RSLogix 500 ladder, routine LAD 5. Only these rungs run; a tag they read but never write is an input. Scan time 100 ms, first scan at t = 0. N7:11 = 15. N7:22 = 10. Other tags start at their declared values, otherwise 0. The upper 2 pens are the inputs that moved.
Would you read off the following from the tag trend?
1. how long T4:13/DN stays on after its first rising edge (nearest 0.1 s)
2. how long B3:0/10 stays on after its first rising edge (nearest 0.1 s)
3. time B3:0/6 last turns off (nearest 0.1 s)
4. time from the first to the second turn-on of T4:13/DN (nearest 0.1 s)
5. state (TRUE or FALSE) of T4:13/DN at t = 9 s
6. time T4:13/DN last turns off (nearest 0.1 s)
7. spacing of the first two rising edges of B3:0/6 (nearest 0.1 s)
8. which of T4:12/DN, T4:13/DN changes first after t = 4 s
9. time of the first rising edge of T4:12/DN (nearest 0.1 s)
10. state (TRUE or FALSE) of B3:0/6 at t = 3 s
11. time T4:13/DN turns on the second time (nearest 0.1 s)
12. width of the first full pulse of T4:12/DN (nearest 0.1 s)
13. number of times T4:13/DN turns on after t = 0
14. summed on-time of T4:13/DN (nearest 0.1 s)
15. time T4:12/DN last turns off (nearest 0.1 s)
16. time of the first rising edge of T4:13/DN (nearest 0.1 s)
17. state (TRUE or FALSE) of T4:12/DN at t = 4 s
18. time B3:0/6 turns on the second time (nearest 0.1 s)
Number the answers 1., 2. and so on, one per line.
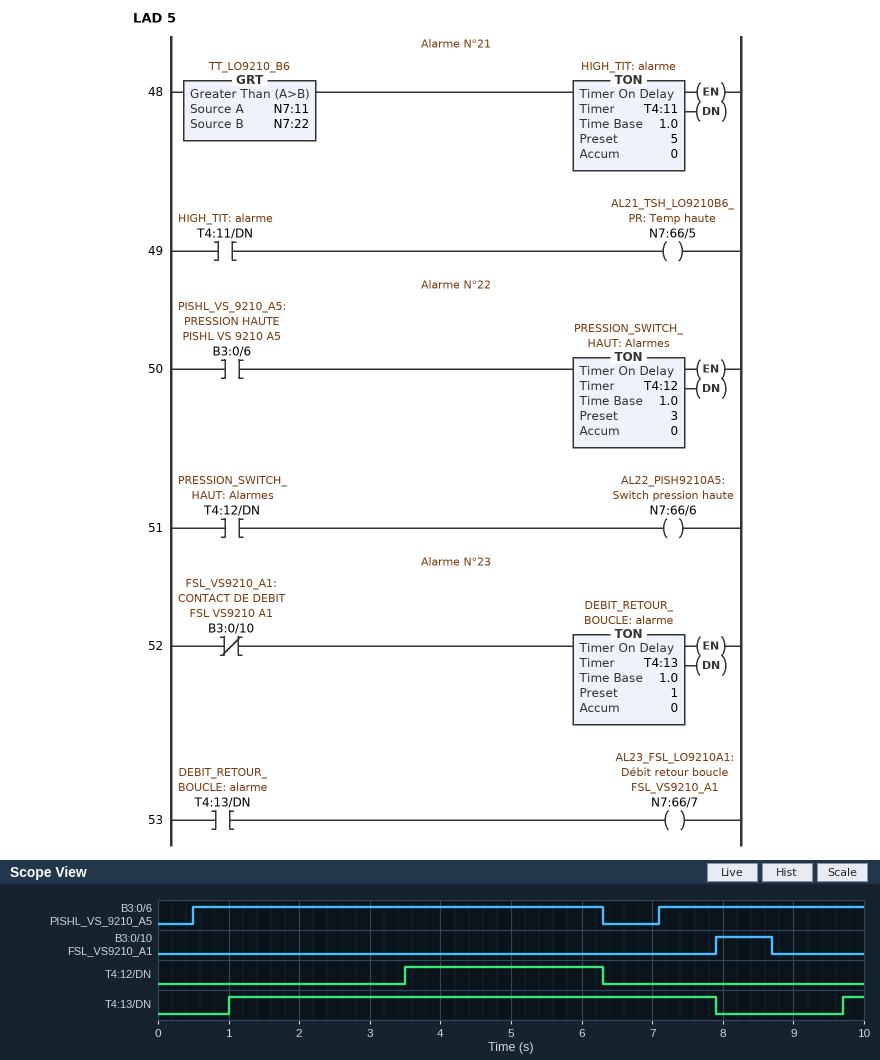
1. 6.9 s
2. 0.8 s
3. 6.3 s
4. 8.7 s
5. FALSE
6. 7.9 s
7. 6.6 s
8. T4:12/DN
9. 3.5 s
10. TRUE
11. 9.7 s
12. 2.8 s
13. 2
14. 7.2 s
15. 6.3 s
16. 1.0 s
17. TRUE
18. 7.1 s
